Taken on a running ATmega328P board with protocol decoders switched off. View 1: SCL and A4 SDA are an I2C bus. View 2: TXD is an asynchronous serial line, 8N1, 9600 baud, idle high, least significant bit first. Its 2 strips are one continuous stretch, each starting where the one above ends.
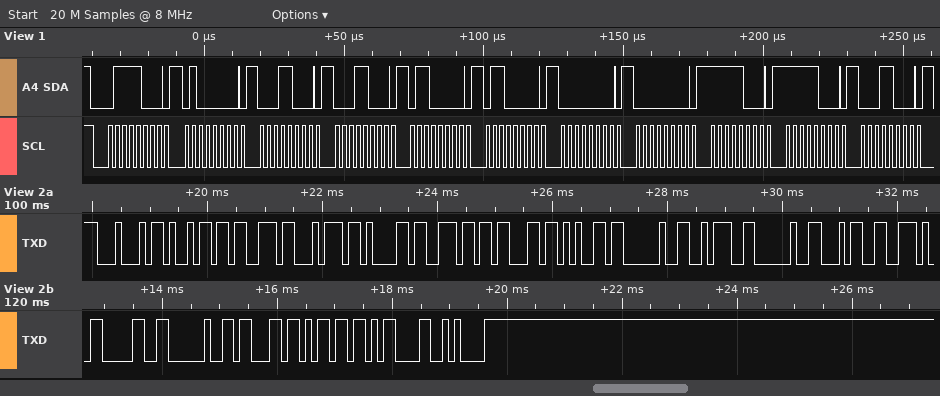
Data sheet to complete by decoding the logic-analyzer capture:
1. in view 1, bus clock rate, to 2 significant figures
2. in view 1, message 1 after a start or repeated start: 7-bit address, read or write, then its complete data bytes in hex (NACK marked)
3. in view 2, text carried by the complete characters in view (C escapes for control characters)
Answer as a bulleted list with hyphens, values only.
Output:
- 400 kHz
- 0x3C write: 40 18 18 60 60 00 00 F8 F8 18
- "Distance : 4.0 cm\r\n"
